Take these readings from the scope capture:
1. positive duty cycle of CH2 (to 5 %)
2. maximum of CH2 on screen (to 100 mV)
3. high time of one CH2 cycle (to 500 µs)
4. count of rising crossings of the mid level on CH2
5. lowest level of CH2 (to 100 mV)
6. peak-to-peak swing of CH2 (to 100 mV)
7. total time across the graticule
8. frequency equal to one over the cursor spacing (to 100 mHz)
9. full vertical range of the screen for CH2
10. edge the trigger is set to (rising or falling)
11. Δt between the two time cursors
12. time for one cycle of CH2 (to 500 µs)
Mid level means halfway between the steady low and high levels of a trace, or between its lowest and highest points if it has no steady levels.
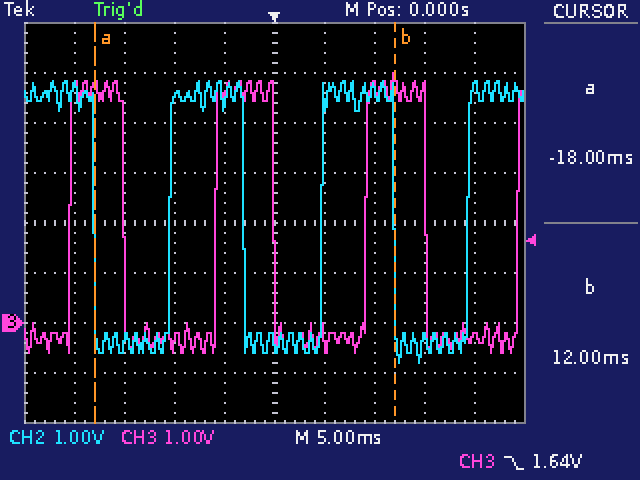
50 %
4.8 V
7.5 ms
3
-800 mV
5.6 V
50 ms
33.3 Hz
8 V
falling
30.0 ms
15.0 ms
